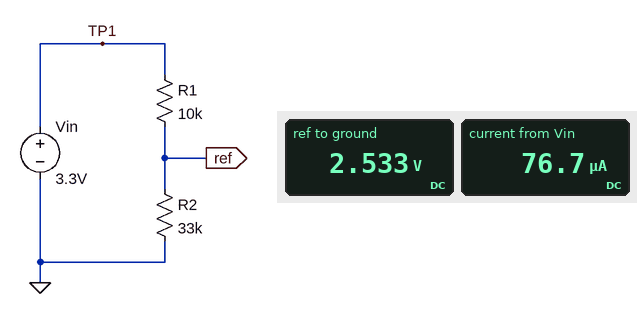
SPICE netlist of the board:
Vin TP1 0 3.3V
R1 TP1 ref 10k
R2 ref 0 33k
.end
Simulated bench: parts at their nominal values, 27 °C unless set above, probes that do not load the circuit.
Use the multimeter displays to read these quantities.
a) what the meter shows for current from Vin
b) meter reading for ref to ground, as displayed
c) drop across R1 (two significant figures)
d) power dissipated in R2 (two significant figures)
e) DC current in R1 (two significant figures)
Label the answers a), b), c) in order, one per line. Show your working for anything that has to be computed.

a) 76.7 µA
b) 2.533 V
c) 3.3 V - 2.533 V = 770 mV
d) (2.533 V)^2 / 33 kΩ = 190 µW
e) (3.3 V - 2.533 V) / 10 kΩ = 77 µA
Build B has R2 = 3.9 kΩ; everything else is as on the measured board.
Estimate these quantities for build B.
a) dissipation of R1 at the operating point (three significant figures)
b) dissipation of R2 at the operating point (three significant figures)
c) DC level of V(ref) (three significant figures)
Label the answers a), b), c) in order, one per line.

a) 564 µW
b) 220 µW
c) 926 mV
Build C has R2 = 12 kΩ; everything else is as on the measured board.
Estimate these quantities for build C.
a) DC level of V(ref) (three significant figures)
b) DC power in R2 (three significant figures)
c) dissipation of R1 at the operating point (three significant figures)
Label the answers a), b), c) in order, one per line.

a) 1.80 V
b) 270 µW
c) 225 µW
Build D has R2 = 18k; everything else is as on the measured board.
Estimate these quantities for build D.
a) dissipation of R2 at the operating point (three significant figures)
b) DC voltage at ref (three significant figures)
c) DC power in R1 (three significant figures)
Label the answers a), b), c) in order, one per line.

a) 250 µW
b) 2.12 V
c) 139 µW
